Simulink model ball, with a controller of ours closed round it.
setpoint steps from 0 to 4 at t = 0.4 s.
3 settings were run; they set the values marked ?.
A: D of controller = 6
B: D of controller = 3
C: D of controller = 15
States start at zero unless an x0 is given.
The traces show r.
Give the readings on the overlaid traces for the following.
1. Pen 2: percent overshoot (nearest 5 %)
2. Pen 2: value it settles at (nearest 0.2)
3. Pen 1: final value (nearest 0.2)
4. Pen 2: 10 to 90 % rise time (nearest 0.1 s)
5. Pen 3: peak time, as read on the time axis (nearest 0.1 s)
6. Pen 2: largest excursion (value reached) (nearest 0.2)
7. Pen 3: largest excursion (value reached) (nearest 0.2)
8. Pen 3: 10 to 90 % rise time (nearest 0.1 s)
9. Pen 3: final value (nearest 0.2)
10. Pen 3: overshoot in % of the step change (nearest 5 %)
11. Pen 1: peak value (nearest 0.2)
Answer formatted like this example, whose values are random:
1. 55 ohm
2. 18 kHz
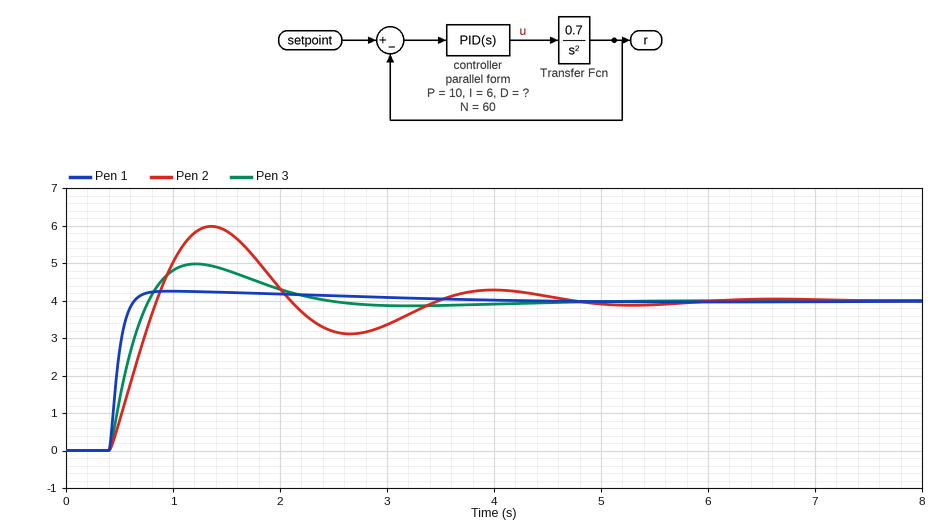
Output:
1. 50 %
2. 4.0
3. 4.0
4. 0.3 s
5. 1.2 s
6. 6.0
7. 5.0
8. 0.3 s
9. 4.0
10. 25 %
11. 4.2
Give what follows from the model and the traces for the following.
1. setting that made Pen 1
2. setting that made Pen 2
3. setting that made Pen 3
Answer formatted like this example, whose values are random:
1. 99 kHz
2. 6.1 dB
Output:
1. C
2. B
3. A
